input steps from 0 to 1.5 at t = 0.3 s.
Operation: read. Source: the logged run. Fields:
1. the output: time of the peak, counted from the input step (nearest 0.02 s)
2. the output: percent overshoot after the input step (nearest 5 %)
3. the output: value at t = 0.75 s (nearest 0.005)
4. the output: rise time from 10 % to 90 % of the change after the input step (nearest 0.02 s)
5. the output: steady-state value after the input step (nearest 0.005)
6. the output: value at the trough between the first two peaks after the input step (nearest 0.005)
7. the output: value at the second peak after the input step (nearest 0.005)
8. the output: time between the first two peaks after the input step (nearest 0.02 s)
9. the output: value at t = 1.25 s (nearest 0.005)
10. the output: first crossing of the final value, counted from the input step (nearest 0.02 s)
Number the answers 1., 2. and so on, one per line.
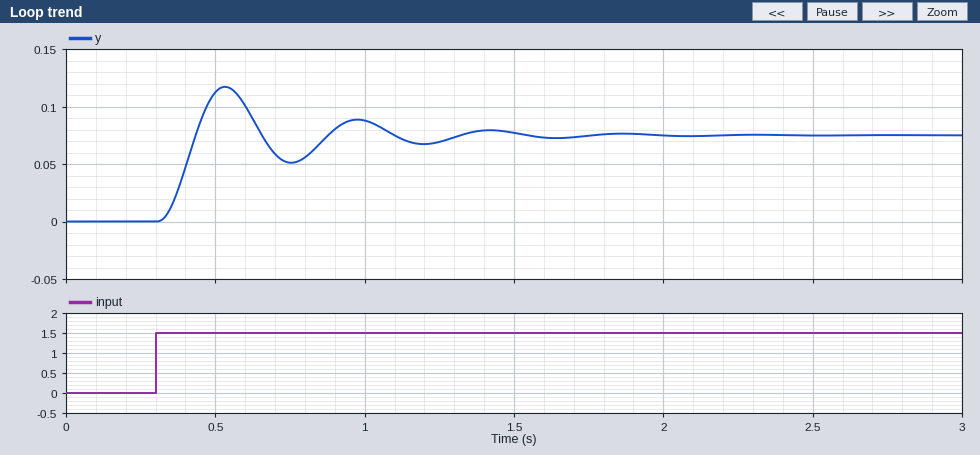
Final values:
1. 0.24 s
2. 55 %
3. 0.050
4. 0.08 s
5. 0.075
6. 0.050
7. 0.090
8. 0.44 s
9. 0.070
10. 0.14 s
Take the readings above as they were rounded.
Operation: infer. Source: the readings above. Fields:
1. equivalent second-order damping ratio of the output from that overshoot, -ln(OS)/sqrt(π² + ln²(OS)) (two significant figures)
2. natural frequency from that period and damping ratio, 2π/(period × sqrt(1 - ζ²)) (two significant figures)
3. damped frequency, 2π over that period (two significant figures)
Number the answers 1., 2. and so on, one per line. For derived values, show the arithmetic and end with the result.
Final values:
1. ln(0.55) = -0.598; 0.598 / sqrt(9.870 + 0.357) = 0.19
2. 2π / (0.44 × sqrt(1 - 0.19²)) = 15 rad/s
3. 2π / 0.44 = 14 rad/s
